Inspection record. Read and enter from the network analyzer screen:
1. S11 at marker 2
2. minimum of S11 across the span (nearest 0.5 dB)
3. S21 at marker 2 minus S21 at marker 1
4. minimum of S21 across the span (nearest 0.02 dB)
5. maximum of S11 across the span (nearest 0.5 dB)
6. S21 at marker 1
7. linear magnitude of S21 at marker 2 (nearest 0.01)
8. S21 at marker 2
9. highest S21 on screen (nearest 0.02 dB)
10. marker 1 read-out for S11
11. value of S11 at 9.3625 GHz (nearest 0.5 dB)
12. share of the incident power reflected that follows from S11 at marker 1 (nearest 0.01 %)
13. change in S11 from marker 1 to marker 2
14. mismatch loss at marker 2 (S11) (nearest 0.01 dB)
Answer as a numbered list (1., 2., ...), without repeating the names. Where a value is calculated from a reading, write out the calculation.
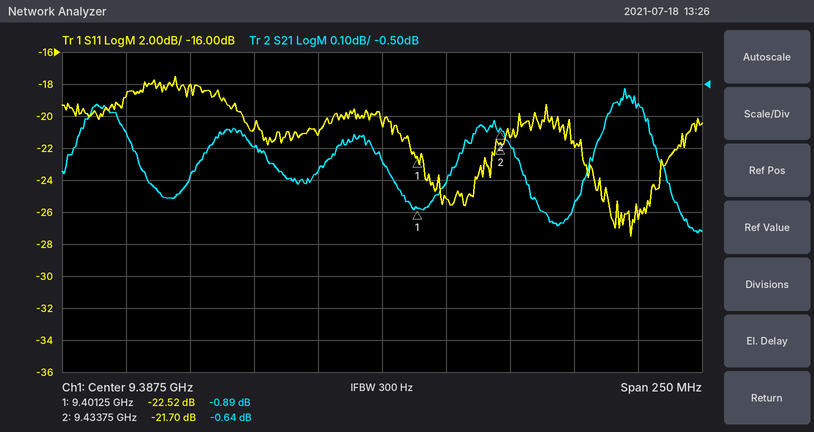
1. -21.70 dB
2. -27.5 dB
3. -0.64 − (-0.89) = 0.25 dB
4. -0.96 dB
5. -17.5 dB
6. -0.89 dB
7. 10^(-0.64/20) ≈ 0.93
8. -0.64 dB
9. -0.52 dB
10. -22.52 dB
11. -21.0 dB
12. 10^(-22.52/10) ≈ 0.56 %
13. -21.7 − (-22.52) = 0.82 dB
14. −10 log10(1 − 10^(-21.7/10)) ≈ 0.03 dB
